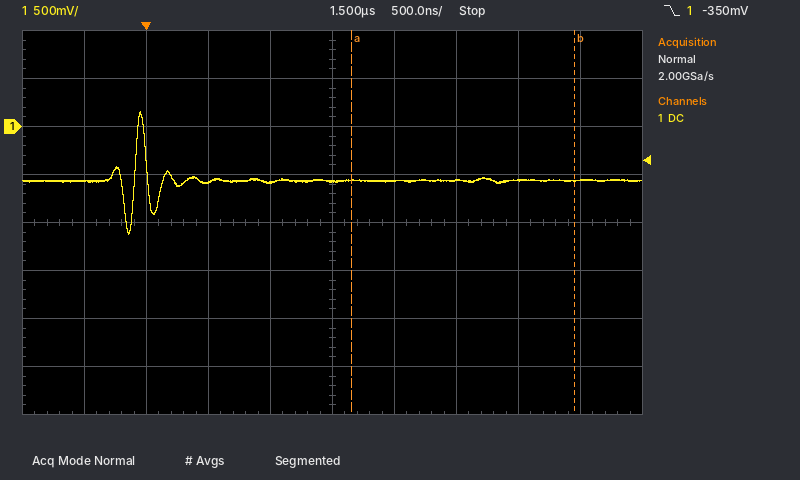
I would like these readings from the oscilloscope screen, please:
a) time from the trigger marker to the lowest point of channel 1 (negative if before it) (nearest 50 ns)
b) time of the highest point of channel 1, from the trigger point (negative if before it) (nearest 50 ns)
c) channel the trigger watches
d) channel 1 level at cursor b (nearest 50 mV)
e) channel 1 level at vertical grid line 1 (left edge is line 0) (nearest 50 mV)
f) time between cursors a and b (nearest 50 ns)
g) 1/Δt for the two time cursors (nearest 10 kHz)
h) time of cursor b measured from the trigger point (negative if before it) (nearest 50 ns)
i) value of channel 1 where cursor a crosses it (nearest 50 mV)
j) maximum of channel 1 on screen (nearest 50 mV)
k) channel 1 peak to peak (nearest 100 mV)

-150 ns
-50 ns
channel 1
-550 mV
-550 mV
1.80 µs
560 kHz
+3.45 µs
-550 mV
150 mV
1.30 V
